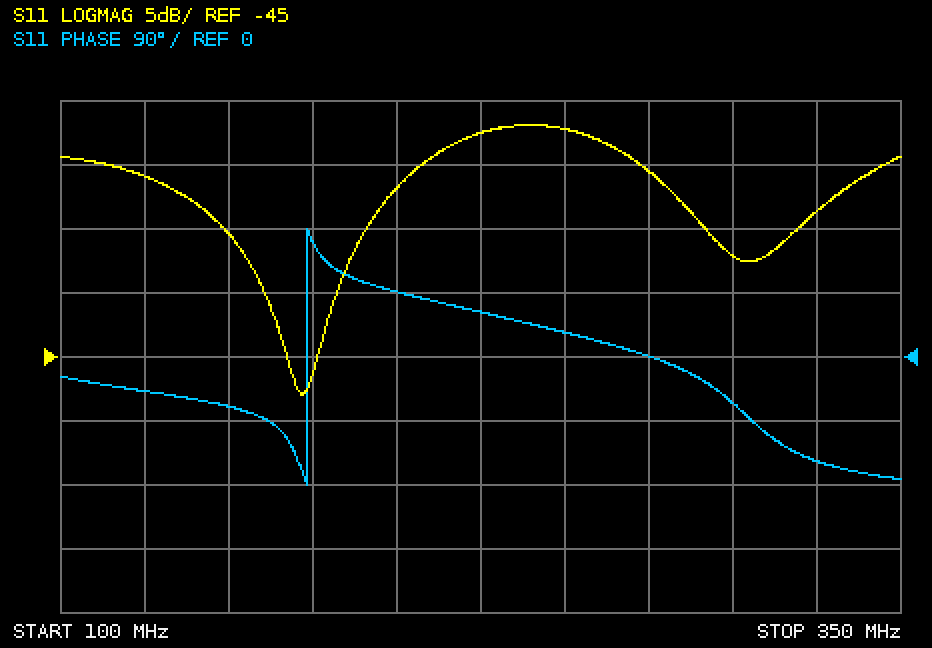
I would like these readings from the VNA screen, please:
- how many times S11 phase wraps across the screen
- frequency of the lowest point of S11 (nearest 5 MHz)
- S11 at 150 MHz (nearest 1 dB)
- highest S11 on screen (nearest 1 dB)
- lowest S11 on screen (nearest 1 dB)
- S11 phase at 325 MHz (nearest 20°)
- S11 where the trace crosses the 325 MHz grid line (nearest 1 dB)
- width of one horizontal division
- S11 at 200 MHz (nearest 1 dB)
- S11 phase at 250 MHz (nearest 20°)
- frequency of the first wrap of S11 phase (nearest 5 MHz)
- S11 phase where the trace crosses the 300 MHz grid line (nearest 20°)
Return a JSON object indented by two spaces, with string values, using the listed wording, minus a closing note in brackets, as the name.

{
  "how many times S11 phase wraps across the screen": "1",
  "frequency of the lowest point of S11": "170 MHz",
  "S11 at 150 MHz": "-35 dB",
  "highest S11 on screen": "-27 dB",
  "lowest S11 on screen": "-48 dB",
  "S11 phase at 325 MHz": "-140°",
  "S11 where the trace crosses the 325 MHz grid line": "-34 dB",
  "width of one horizontal division": "25 MHz",
  "S11 at 200 MHz": "-32 dB",
  "S11 phase at 250 MHz": "40°",
  "frequency of the first wrap of S11 phase": "175 MHz",
  "S11 phase where the trace crosses the 300 MHz grid line": "-60°"
}
